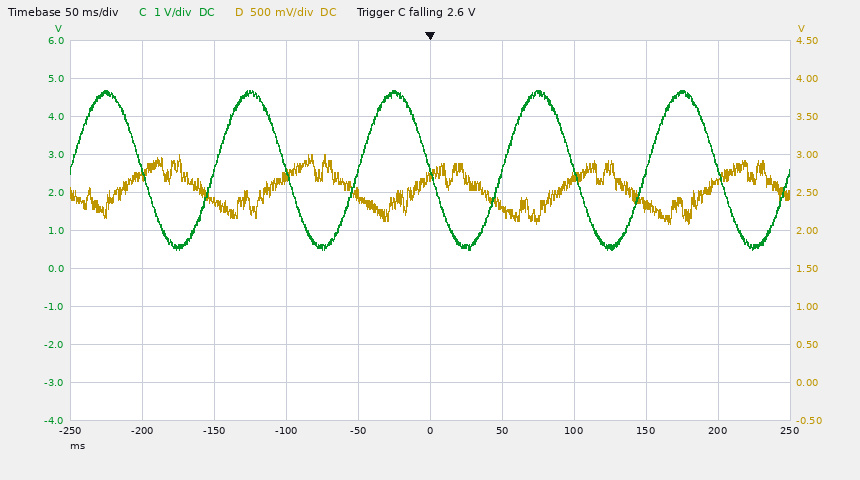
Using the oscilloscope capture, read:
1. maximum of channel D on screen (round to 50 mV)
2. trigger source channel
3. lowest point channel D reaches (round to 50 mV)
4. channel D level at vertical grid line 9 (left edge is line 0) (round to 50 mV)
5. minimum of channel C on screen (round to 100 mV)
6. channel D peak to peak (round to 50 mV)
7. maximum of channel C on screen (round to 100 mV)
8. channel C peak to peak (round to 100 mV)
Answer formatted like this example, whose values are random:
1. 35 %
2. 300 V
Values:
1. 3.00 V
2. channel C
3. 2.10 V
4. 2.65 V
5. 500 mV
6. 900 mV
7. 4.7 V
8. 4.2 V
